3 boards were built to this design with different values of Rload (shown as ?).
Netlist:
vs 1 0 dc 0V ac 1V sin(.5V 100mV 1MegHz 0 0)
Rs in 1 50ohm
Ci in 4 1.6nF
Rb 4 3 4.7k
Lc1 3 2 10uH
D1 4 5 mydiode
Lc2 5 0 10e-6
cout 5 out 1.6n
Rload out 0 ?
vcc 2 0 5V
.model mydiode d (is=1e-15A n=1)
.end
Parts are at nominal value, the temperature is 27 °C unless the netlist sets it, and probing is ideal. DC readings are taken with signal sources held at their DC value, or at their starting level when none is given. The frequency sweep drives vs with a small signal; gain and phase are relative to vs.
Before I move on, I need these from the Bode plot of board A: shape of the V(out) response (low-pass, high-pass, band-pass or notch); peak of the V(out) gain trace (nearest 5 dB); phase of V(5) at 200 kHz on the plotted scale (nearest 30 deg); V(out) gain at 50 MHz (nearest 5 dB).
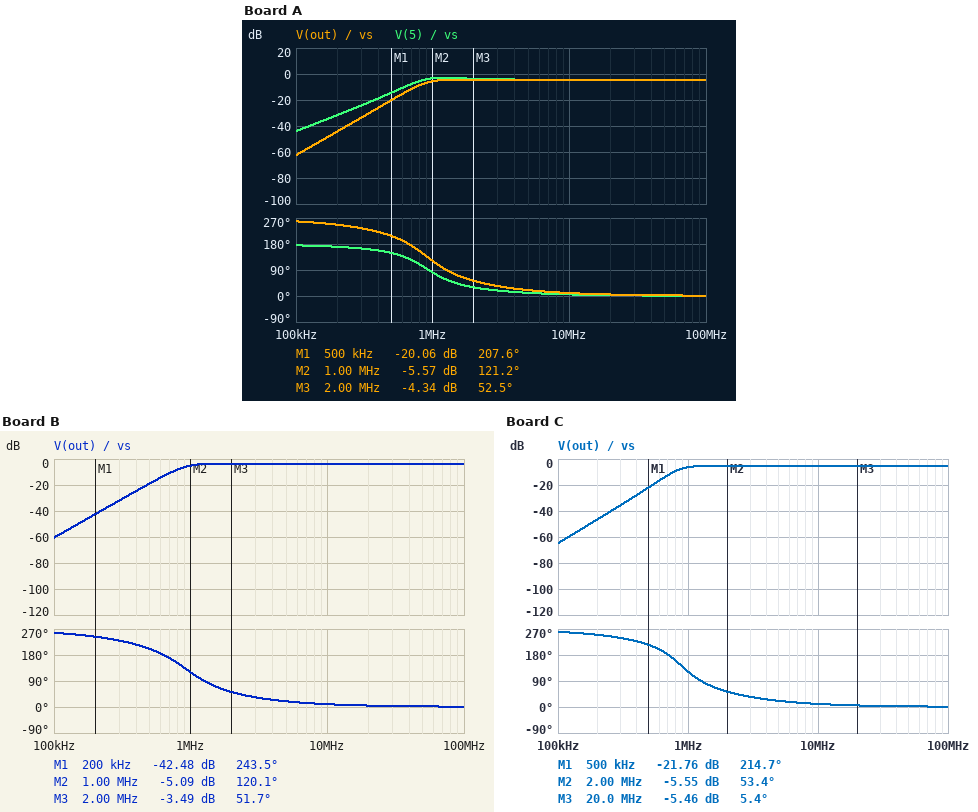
high-pass
-5 dB
180 deg
-5 dB
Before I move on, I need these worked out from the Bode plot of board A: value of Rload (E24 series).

120 Ω
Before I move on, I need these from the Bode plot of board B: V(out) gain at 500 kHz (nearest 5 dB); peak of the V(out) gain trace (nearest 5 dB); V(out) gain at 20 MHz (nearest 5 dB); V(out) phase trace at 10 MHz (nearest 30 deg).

-20 dB
-5 dB
-5 dB
0 deg
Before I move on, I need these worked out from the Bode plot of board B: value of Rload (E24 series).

150 Ω
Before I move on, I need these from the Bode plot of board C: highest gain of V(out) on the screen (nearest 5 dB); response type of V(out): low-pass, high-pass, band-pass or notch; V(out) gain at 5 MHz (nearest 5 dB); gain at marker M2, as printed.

-5 dB
high-pass
-5 dB
-5.55 dB
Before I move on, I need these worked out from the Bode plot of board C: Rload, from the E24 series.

91 Ω
